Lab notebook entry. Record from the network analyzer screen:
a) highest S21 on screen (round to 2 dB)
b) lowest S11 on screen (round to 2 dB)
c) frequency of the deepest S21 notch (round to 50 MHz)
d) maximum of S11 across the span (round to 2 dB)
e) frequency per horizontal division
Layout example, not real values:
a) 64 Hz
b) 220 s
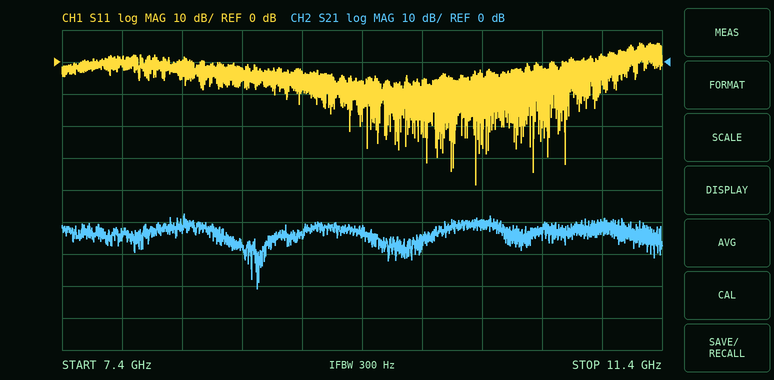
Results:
a) -48 dB
b) -38 dB
c) 8.70 GHz
d) 6 dB
e) 400 MHz
